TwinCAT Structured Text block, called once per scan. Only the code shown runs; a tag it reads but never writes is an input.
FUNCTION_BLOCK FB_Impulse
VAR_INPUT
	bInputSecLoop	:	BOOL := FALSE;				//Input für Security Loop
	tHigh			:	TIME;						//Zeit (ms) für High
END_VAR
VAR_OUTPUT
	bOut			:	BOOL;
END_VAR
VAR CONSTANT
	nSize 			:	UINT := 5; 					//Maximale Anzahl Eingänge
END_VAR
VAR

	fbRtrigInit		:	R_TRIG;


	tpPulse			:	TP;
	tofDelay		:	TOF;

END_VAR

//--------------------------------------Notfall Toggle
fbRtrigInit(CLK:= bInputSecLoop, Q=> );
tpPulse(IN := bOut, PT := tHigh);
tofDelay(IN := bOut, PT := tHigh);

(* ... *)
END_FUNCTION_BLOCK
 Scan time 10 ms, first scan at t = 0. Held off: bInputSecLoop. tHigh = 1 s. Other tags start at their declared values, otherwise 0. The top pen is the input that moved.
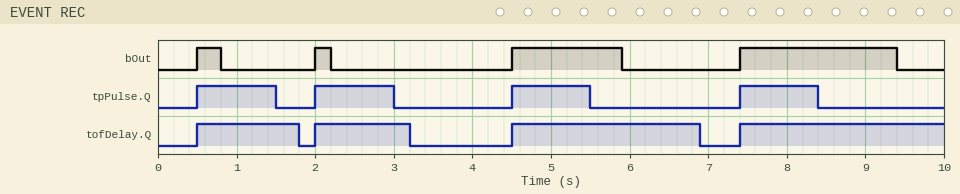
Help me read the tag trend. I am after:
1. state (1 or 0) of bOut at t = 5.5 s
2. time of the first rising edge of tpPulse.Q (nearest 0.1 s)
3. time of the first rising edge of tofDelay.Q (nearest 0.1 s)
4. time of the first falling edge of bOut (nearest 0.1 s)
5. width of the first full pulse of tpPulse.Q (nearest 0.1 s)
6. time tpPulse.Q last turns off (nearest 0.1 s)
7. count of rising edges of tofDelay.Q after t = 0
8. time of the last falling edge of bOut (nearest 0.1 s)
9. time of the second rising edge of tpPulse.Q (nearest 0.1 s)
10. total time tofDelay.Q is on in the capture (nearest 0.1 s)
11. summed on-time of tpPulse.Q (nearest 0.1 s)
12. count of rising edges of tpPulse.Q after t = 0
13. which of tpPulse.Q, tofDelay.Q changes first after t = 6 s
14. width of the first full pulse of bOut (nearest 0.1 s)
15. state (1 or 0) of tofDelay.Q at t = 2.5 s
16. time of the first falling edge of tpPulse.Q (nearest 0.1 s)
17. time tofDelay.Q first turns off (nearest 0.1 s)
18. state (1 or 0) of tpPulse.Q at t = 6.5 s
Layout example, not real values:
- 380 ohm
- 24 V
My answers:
- 1
- 0.5 s
- 0.5 s
- 0.8 s
- 1.0 s
- 8.4 s
- 4
- 9.4 s
- 2.0 s
- 7.5 s
- 4.0 s
- 4
- tofDelay.Q
- 0.3 s
- 1
- 1.5 s
- 1.8 s
- 0
